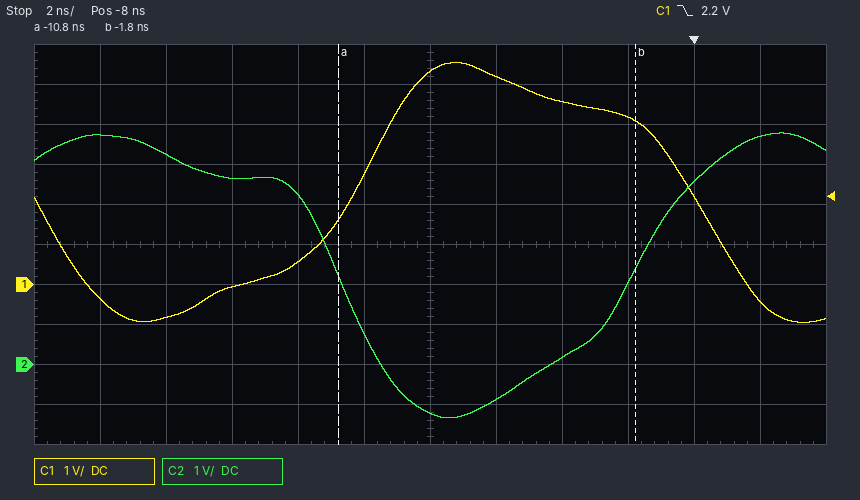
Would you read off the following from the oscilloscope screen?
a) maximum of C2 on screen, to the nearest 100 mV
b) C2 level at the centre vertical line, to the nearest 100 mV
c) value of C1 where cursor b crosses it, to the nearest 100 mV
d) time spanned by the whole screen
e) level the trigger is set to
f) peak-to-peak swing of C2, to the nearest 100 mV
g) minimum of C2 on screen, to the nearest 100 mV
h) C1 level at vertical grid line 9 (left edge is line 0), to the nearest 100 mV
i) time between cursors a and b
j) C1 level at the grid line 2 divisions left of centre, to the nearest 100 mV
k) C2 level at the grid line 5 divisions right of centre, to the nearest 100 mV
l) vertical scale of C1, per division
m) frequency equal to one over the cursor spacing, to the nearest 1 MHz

5.8 V
-1.2 V
4.1 V
24 ns
2.2 V
7.1 V
-1.3 V
4.2 V
9.0 ns
600 mV
5.7 V
1 V
111 MHz
